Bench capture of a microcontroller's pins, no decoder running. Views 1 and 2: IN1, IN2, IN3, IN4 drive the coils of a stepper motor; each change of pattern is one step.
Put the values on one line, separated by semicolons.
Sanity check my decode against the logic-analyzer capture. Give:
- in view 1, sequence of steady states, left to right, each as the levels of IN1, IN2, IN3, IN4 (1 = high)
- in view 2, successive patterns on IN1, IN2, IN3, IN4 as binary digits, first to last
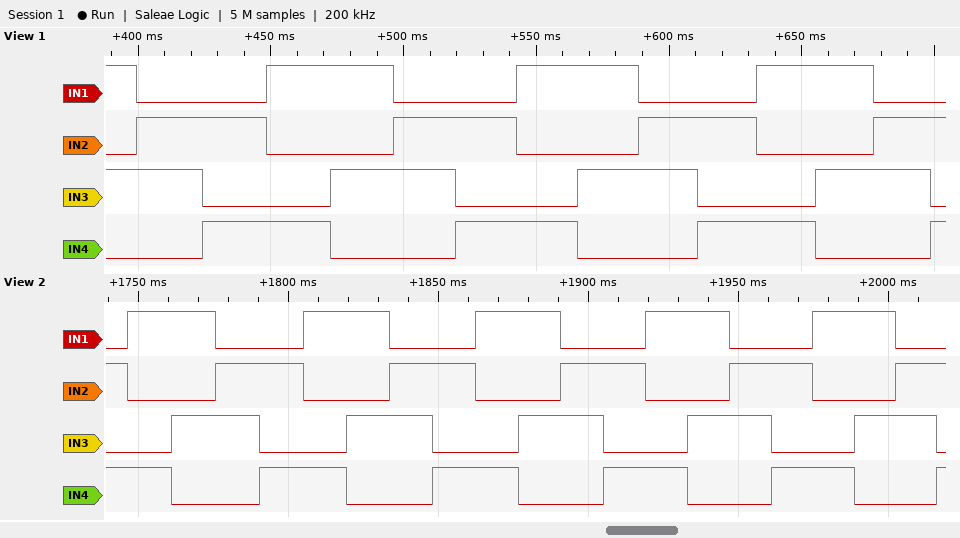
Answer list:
1010 0110 0101 1001 1010 0110 0101 1001 1010 0110 0101 1001 1010 0110 0101; 0101 1001 1010 0110 0101 1001 1010 0110 0101 1001 1010 0110 0101 1001 1010 0110 0101 1001 1010 0110 0101
